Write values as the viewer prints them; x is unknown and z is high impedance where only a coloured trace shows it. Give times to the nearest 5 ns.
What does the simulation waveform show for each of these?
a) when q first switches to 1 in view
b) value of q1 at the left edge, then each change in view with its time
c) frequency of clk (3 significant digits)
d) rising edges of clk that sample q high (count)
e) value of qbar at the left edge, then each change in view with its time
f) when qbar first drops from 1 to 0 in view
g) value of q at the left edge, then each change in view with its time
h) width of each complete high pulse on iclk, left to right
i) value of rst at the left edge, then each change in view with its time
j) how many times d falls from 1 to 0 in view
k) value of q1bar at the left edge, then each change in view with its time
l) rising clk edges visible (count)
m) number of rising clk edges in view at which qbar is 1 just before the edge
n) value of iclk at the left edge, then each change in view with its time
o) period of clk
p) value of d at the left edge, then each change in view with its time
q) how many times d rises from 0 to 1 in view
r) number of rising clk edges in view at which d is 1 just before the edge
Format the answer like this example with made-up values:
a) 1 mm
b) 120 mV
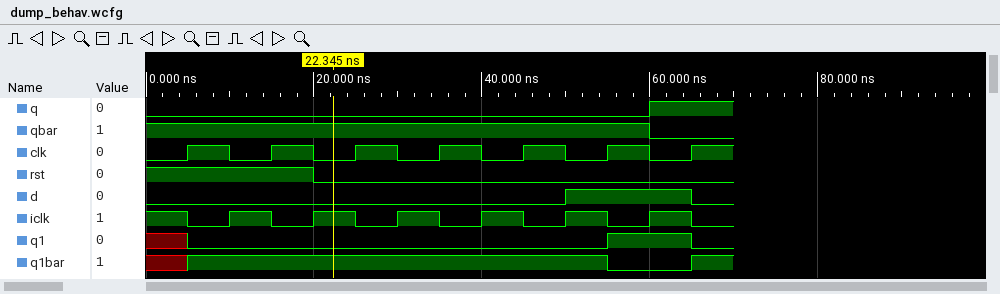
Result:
a) 60 ns
b) x, 0 at 5 ns, 1 at 55 ns, 0 at 65 ns
c) 100 MHz
d) 1
e) 1, 0 at 60 ns
f) 60 ns
g) 0, 1 at 60 ns
h) 5 ns, 5 ns, 5 ns, 5 ns, 5 ns, 5 ns
i) 1, 0 at 20 ns
j) 1
k) x, 1 at 5 ns, 0 at 55 ns, 1 at 65 ns
l) 7
m) 6
n) 1, 0 at 5 ns, 1 at 10 ns, 0 at 15 ns, 1 at 20 ns, 0 at 25 ns, 1 at 30 ns, 0 at 35 ns, 1 at 40 ns, 0 at 45 ns, 1 at 50 ns, 0 at 55 ns, 1 at 60 ns, 0 at 65 ns
o) 10 ns
p) 0, 1 at 50 ns, 0 at 65 ns
q) 1
r) 2
